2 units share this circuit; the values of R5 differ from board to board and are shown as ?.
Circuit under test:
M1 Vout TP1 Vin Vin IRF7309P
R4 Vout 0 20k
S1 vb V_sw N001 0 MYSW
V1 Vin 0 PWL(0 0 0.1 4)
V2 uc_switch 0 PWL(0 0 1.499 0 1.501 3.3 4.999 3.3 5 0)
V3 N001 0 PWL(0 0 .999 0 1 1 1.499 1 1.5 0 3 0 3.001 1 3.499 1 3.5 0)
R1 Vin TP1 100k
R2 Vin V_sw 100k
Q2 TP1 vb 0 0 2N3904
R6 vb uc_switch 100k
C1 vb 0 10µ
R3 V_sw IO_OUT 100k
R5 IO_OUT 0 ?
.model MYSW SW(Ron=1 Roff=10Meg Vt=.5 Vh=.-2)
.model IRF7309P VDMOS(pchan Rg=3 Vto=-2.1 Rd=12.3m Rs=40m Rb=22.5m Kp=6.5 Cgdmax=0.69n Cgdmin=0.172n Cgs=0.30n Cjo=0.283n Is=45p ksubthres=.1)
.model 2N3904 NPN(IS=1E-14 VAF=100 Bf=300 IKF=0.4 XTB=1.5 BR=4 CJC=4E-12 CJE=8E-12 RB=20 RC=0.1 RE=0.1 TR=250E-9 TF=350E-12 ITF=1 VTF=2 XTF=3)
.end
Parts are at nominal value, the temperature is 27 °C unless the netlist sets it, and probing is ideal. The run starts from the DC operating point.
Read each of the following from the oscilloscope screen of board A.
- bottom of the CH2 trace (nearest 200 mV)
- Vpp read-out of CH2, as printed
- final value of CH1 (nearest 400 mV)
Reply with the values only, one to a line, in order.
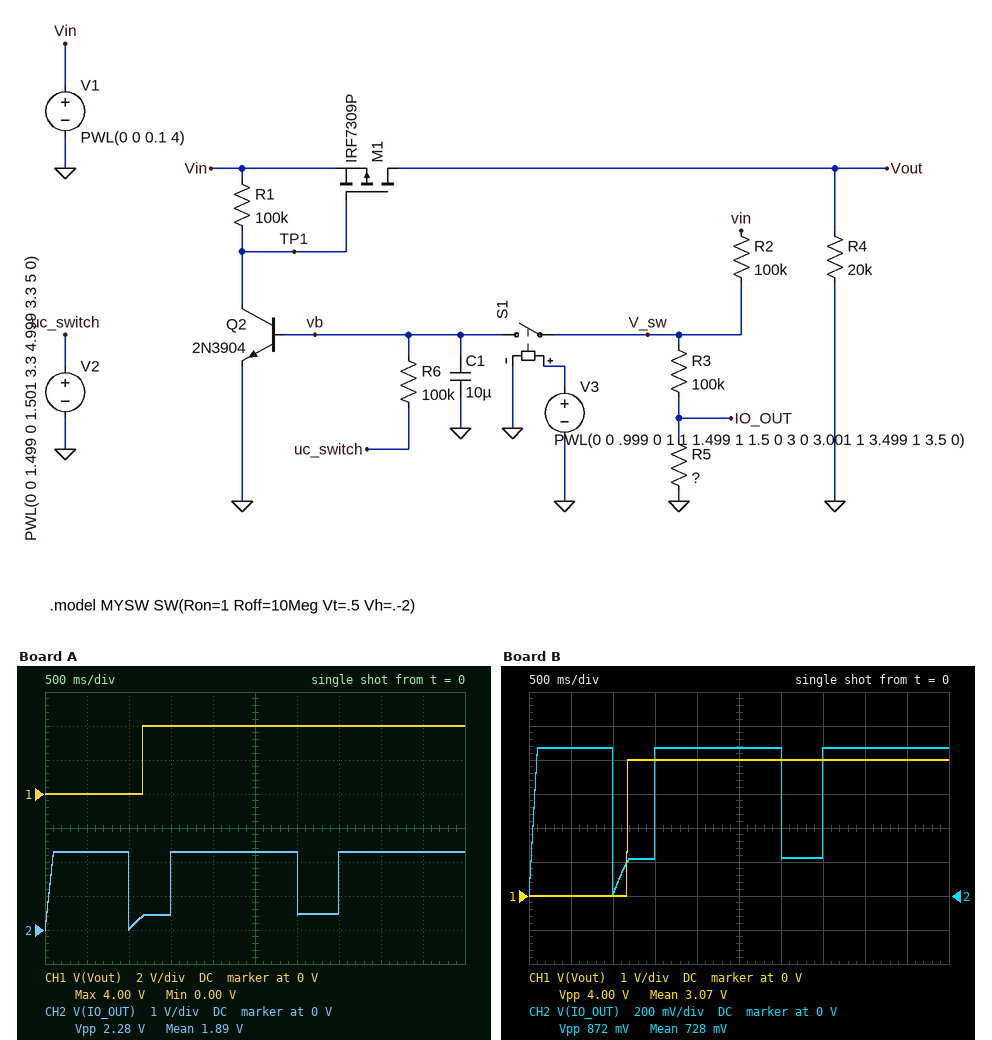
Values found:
0 V
2.28 V
4.0 V
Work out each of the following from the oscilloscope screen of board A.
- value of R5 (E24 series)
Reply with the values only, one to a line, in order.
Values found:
270 kΩ
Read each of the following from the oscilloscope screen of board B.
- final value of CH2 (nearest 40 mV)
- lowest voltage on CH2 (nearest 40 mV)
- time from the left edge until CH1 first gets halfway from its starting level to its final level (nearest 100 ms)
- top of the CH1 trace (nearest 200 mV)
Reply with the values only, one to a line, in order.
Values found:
880 mV
0 V
1.2 s
4.0 V
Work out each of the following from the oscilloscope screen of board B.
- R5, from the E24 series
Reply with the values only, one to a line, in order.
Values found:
56 kΩ
